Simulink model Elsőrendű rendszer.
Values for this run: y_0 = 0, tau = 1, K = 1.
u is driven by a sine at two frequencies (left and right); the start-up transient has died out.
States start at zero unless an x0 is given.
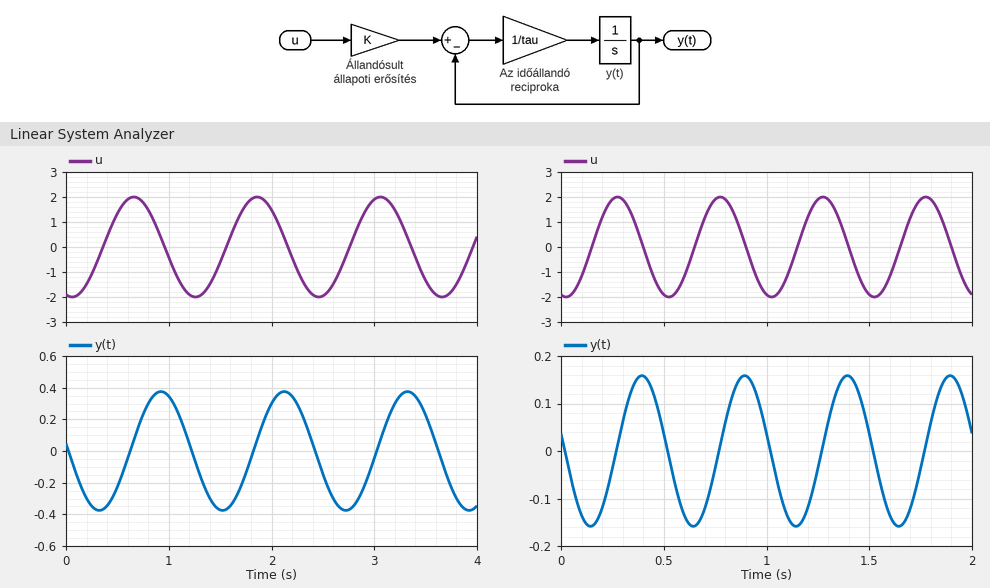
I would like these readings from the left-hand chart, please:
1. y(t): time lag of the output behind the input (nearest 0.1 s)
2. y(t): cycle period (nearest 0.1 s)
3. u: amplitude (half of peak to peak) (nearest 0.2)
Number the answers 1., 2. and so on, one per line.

1. 0.3 s
2. 1.2 s
3. 2.0
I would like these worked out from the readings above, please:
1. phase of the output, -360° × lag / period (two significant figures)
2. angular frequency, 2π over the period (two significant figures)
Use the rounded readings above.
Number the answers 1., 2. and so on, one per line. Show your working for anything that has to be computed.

1. -360 × 0.3 / 1.2 = -90°
2. 2π / 1.2 = 5.2 rad/s
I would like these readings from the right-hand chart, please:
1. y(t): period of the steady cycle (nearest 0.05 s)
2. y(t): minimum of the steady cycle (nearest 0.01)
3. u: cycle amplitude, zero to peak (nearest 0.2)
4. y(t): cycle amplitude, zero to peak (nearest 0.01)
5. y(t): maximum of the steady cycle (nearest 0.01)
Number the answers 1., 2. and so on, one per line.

1. 0.50 s
2. -0.16
3. 2.0
4. 0.16
5. 0.16
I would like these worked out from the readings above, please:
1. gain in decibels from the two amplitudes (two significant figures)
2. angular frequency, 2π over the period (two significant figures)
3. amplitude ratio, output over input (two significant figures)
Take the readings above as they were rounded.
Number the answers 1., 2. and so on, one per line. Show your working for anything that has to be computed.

1. 20 log10(0.16 / 2) = -22 dB
2. 2π / 0.5 = 13 rad/s
3. 0.16 / 2 = 0.080
